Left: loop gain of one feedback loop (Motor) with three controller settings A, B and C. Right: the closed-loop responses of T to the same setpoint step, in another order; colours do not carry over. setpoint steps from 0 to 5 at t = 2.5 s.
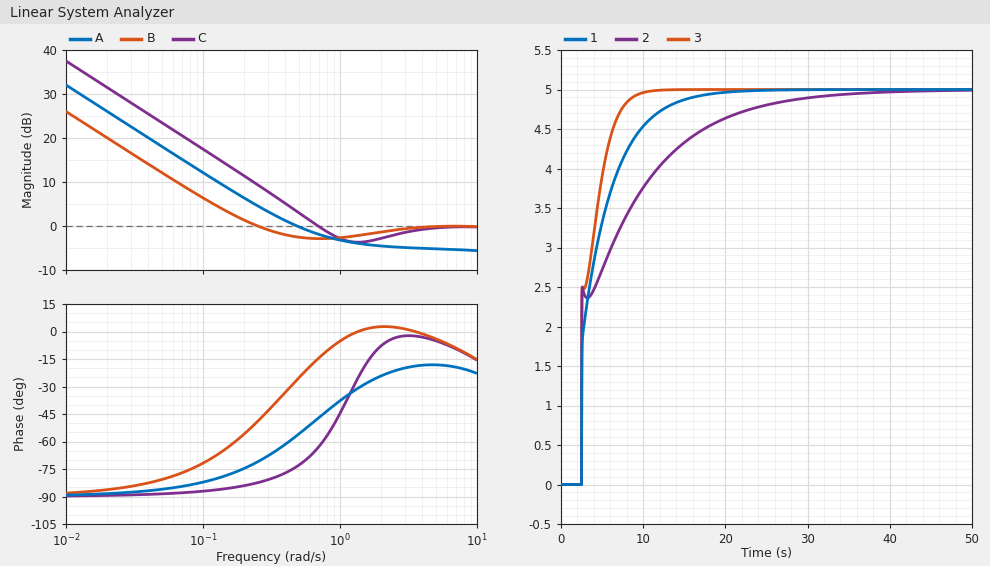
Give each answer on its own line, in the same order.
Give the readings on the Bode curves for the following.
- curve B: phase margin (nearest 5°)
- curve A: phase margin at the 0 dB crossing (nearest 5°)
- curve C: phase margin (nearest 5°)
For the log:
130°
125°
115°
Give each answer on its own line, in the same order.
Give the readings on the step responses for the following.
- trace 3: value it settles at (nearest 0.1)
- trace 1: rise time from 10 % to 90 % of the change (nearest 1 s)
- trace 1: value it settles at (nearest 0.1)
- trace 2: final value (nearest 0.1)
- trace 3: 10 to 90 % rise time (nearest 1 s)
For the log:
5.0
7 s
5.0
5.0
4 s
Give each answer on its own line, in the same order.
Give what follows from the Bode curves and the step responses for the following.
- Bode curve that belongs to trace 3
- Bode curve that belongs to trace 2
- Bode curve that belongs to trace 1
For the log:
C
B
A
